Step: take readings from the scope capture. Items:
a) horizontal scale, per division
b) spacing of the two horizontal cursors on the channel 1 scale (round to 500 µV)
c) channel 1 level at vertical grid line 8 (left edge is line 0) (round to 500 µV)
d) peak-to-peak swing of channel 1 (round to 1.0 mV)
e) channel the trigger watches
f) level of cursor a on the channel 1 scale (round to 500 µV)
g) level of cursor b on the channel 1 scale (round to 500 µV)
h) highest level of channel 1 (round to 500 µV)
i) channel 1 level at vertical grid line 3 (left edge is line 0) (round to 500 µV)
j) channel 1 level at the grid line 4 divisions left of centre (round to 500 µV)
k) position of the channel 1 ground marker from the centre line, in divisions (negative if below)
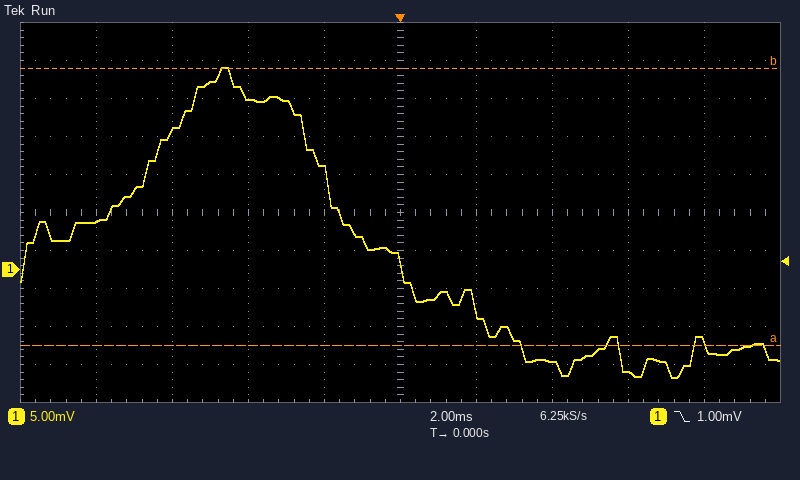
2 ms
36.5 mV
-13.5 mV
41.0 mV
channel 1
-10.0 mV
26.5 mV
26.5 mV
22.5 mV
6.5 mV
-1.5 div
